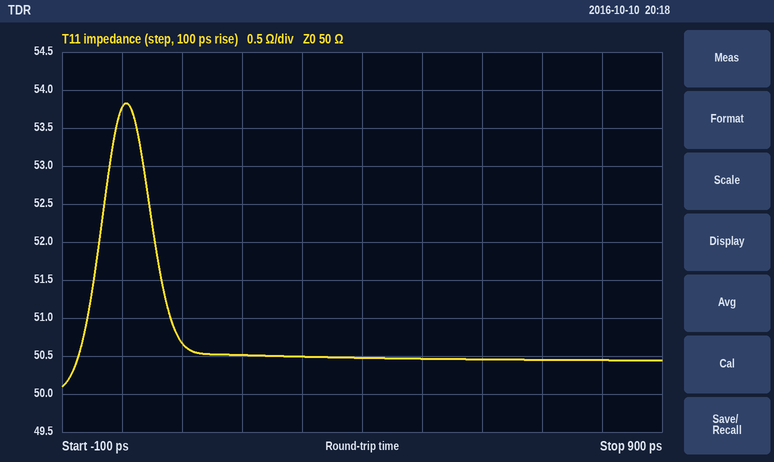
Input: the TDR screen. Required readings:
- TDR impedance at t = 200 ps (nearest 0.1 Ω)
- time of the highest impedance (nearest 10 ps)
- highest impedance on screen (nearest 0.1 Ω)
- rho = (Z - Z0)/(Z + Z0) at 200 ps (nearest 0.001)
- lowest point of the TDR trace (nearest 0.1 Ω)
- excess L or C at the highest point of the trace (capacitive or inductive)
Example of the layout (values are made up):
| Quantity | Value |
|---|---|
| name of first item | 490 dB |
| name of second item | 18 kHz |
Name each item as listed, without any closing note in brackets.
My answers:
| Quantity | Value |
|---|---|
| TDR impedance at t = 200 ps | 50.5 Ω |
| time of the highest impedance | 10 ps |
| highest impedance on screen | 53.8 Ω |
| rho = (Z - Z0)/(Z + Z0) at 200 ps | +0.005 |
| lowest point of the TDR trace | 50.1 Ω |
| excess L or C at the highest point of the trace | inductive |
